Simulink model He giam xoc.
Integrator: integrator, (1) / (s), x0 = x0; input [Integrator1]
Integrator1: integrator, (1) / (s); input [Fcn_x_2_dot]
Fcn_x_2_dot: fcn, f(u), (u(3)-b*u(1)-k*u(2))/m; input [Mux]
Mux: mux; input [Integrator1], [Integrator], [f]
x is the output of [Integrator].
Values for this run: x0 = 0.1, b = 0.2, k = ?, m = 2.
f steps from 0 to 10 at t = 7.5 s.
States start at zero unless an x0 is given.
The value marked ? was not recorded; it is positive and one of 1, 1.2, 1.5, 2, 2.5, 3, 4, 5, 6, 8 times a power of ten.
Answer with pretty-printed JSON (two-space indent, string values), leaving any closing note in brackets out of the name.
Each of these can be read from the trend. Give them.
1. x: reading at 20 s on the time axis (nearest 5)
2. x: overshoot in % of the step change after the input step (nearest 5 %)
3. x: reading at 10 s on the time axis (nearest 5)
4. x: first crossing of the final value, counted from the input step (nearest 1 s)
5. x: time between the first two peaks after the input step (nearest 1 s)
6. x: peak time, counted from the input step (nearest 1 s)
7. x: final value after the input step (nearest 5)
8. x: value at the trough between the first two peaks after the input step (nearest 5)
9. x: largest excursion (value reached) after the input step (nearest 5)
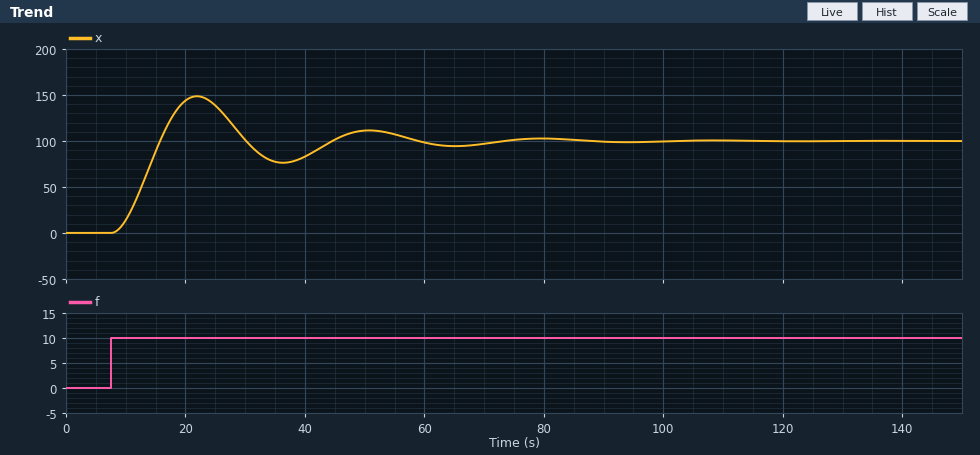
{
  "x: reading at 20 s on the time axis": "145",
  "x: overshoot in % of the step change after the input step": "50 %",
  "x: reading at 10 s on the time axis": "15",
  "x: first crossing of the final value, counted from the input step": "8 s",
  "x: time between the first two peaks after the input step": "29 s",
  "x: peak time, counted from the input step": "14 s",
  "x: final value after the input step": "100",
  "x: value at the trough between the first two peaks after the input step": "75",
  "x: largest excursion (value reached) after the input step": "150"
}
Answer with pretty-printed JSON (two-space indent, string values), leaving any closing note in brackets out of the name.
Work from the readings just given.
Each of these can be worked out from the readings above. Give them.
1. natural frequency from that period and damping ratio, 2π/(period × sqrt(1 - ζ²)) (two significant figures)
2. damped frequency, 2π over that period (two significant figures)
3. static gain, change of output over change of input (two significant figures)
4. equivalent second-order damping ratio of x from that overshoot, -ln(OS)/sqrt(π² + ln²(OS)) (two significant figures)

{
  "natural frequency from that period and damping ratio, 2π/(period × sqrt(1 - ζ²))": "0.22 rad/s",
  "damped frequency, 2π over that period": "0.22 rad/s",
  "static gain, change of output over change of input": "10",
  "equivalent second-order damping ratio of x from that overshoot, -ln(OS)/sqrt(π² + ln²(OS))": "0.22"
}
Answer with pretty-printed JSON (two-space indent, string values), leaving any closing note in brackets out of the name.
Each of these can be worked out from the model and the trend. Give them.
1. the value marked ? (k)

{
  "the value marked ?": "0.1"
}
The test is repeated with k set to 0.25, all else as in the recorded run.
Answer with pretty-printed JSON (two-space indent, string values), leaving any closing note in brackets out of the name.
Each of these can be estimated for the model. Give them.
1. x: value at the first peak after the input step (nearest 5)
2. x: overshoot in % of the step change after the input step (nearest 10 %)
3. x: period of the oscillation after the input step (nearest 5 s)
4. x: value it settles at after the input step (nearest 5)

{
  "x: value at the first peak after the input step": "65",
  "x: overshoot in % of the step change after the input step": "60 %",
  "x: period of the oscillation after the input step": "20 s",
  "x: value it settles at after the input step": "40"
}
